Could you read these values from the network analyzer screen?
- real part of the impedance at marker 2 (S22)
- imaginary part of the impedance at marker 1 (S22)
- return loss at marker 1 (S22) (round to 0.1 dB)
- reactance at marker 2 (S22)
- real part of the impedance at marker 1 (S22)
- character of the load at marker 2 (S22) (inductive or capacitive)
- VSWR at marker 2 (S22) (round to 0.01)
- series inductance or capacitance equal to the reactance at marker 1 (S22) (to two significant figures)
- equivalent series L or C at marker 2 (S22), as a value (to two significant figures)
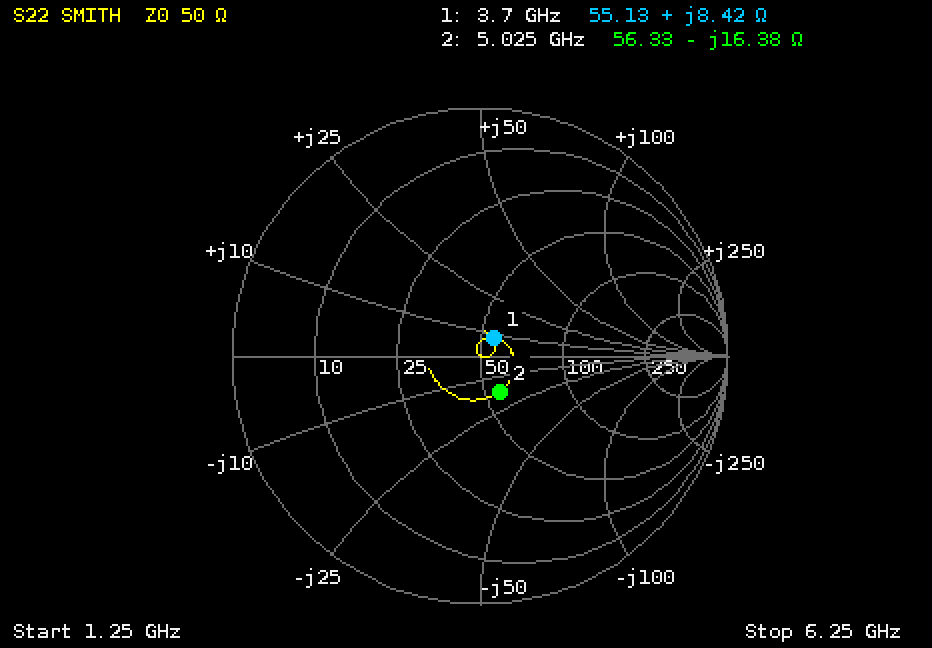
56.33 Ω
+8.42 Ω
20.6 dB
-16.38 Ω
55.13 Ω
capacitive
1.39
360 pH
1.9 pF
